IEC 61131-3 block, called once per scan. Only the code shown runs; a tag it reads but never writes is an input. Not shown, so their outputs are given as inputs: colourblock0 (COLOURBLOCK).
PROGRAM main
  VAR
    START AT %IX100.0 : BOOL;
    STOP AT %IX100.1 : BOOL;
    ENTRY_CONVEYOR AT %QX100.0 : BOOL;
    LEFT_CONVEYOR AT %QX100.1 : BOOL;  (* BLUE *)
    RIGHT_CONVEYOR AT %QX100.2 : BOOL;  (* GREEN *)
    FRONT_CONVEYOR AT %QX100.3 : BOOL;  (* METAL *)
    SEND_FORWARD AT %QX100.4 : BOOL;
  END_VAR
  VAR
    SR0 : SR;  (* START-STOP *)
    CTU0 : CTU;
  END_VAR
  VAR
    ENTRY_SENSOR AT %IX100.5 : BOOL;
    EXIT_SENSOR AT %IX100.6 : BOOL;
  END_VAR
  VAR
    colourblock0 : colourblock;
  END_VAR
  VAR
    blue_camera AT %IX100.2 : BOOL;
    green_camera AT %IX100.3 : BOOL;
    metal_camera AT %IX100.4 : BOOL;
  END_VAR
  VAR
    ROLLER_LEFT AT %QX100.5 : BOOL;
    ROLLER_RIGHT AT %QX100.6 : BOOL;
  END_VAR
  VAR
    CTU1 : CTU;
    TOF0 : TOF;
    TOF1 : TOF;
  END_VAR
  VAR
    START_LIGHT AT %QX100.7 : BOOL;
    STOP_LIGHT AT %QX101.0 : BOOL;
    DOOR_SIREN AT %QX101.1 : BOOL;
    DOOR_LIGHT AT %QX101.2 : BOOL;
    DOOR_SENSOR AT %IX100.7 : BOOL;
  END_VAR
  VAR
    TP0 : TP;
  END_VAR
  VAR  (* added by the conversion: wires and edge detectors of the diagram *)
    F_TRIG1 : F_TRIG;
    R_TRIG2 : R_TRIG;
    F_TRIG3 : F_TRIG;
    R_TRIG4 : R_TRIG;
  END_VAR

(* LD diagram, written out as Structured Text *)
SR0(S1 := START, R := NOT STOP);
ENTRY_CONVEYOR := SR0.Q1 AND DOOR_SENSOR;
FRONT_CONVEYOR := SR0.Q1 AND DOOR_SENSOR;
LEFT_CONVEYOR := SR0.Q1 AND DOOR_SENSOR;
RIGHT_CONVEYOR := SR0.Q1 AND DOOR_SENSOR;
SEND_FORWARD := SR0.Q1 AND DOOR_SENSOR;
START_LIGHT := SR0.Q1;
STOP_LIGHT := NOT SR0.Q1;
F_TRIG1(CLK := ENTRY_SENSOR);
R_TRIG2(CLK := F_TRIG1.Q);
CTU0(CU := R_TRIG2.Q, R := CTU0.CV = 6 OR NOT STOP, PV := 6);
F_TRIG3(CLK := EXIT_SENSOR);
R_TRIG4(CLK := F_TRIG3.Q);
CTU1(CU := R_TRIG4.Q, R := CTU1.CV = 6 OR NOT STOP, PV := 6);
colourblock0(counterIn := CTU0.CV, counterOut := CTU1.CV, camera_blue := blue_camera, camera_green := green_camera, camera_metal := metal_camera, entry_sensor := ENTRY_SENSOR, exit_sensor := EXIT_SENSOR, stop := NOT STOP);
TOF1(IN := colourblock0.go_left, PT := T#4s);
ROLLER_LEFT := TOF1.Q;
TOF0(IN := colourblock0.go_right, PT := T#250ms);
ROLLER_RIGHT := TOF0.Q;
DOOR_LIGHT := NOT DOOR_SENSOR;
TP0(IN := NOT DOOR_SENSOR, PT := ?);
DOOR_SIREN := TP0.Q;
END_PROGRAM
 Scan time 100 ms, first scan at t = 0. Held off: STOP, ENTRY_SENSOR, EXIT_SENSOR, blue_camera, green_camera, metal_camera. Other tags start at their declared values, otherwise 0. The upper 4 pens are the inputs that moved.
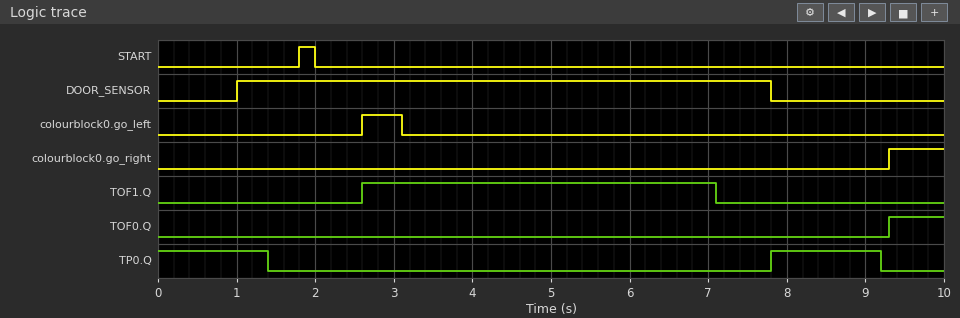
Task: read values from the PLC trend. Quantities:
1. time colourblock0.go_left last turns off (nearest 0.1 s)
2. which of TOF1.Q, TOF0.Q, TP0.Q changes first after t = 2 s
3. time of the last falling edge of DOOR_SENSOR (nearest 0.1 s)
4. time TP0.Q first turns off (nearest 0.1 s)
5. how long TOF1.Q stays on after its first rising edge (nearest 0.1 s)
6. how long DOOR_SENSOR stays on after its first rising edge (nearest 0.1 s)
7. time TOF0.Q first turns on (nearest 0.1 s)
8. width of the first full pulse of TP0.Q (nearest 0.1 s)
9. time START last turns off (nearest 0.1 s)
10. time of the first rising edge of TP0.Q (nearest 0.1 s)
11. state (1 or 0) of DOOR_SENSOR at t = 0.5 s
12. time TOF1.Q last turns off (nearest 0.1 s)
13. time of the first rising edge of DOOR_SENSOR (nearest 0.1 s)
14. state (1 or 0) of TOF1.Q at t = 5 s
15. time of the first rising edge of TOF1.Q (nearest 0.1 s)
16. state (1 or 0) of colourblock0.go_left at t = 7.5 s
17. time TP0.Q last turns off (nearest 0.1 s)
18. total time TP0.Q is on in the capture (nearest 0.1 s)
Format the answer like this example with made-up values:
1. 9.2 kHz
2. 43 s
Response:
1. 3.1 s
2. TOF1.Q
3. 7.8 s
4. 1.4 s
5. 4.5 s
6. 6.8 s
7. 9.3 s
8. 1.4 s
9. 2.0 s
10. 7.8 s
11. 0
12. 7.1 s
13. 1.0 s
14. 1
15. 2.6 s
16. 0
17. 9.2 s
18. 2.8 s
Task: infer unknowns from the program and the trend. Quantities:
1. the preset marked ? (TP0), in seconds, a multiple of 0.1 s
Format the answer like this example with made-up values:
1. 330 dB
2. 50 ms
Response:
1. 1.4 s
